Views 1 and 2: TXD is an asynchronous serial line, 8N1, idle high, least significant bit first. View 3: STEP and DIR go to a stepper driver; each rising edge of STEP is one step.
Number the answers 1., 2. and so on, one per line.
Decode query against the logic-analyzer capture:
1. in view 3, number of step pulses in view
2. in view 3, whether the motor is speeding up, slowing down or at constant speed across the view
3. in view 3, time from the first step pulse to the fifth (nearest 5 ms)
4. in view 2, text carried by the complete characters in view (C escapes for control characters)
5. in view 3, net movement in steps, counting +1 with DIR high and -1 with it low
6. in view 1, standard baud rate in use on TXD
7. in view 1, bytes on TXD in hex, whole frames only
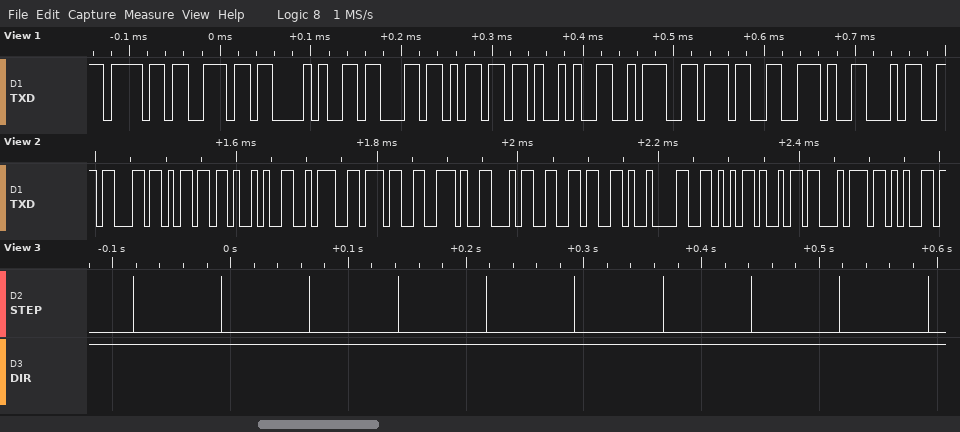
1. 10
2. constant speed
3. 300 ms
4. "cm):7.46\tVite"
5. +10
6. 115200 baud
7. 6F 6E 28 63 6D 29 3A 37 2E 34
